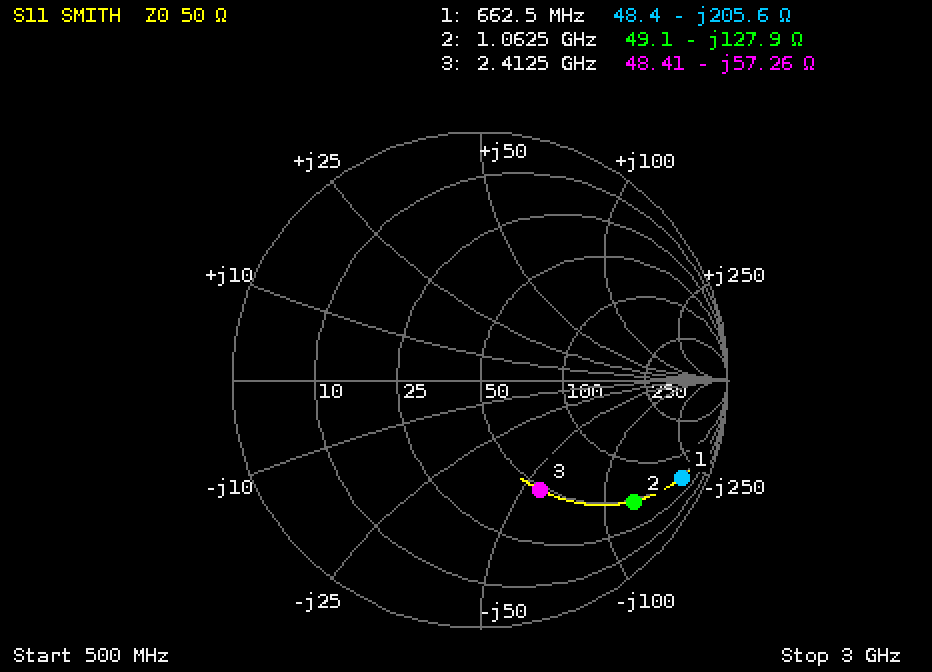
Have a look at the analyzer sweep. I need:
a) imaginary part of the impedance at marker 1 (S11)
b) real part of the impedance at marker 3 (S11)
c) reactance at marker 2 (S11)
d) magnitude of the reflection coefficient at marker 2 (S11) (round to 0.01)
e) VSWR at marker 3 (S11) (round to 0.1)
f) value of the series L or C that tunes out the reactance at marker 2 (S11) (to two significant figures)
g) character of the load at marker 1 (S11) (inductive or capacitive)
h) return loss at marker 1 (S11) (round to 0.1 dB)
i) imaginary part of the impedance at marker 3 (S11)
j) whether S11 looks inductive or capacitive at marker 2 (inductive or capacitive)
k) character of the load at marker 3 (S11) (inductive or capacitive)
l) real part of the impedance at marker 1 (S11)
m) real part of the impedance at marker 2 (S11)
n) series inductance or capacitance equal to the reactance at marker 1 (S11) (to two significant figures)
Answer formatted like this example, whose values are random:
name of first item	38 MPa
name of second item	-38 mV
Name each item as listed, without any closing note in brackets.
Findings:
imaginary part of the impedance at marker 1	-205.6 Ω
real part of the impedance at marker 3	48.41 Ω
reactance at marker 2	-127.9 Ω
magnitude of the reflection coefficient at marker 2 (S11)	0.79
VSWR at marker 3 (S11)	3.0
value of the series L or C that tunes out the reactance at marker 2 (S11)	19 nH
character of the load at marker 1 (S11)	capacitive
return loss at marker 1 (S11)	0.9 dB
imaginary part of the impedance at marker 3	-57.26 Ω
whether S11 looks inductive or capacitive at marker 2	capacitive
character of the load at marker 3 (S11)	capacitive
real part of the impedance at marker 1	48.4 Ω
real part of the impedance at marker 2	49.1 Ω
series inductance or capacitance equal to the reactance at marker 1 (S11)	1.2 pF
